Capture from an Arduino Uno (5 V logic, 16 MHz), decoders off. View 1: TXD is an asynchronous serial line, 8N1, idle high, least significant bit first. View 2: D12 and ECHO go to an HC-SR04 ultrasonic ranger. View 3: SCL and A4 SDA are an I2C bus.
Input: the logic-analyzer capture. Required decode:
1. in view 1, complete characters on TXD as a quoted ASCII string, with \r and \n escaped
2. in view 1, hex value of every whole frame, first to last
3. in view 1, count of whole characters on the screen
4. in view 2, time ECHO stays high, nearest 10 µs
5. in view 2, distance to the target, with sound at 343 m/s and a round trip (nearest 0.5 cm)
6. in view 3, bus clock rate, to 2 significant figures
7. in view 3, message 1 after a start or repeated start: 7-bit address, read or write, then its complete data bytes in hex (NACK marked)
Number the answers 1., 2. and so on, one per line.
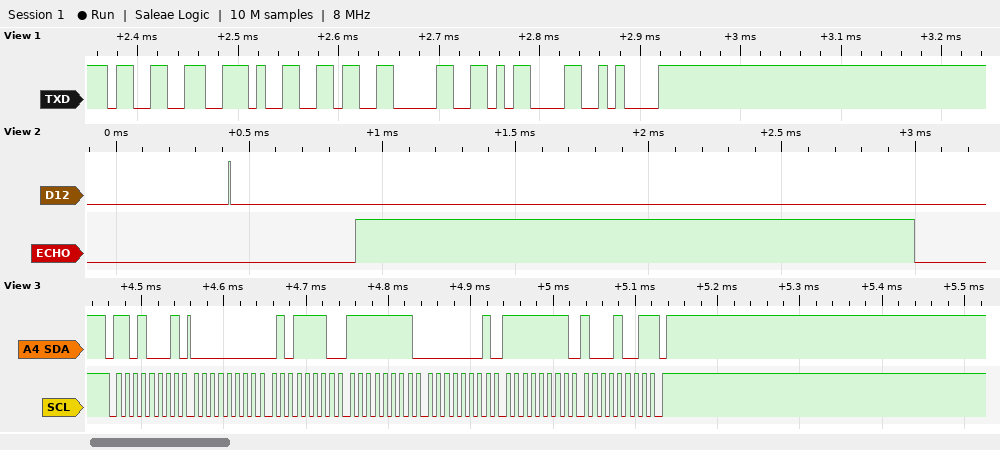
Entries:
1. "3.60\r\n"
2. 0x33 0x2E 0x36 0x30 0x0D 0x0A
3. 6
4. 2100 µs
5. 36 cm
6. 100 kHz
7. 0x68 read: 00 5E FF 01 FF 89 NACK
